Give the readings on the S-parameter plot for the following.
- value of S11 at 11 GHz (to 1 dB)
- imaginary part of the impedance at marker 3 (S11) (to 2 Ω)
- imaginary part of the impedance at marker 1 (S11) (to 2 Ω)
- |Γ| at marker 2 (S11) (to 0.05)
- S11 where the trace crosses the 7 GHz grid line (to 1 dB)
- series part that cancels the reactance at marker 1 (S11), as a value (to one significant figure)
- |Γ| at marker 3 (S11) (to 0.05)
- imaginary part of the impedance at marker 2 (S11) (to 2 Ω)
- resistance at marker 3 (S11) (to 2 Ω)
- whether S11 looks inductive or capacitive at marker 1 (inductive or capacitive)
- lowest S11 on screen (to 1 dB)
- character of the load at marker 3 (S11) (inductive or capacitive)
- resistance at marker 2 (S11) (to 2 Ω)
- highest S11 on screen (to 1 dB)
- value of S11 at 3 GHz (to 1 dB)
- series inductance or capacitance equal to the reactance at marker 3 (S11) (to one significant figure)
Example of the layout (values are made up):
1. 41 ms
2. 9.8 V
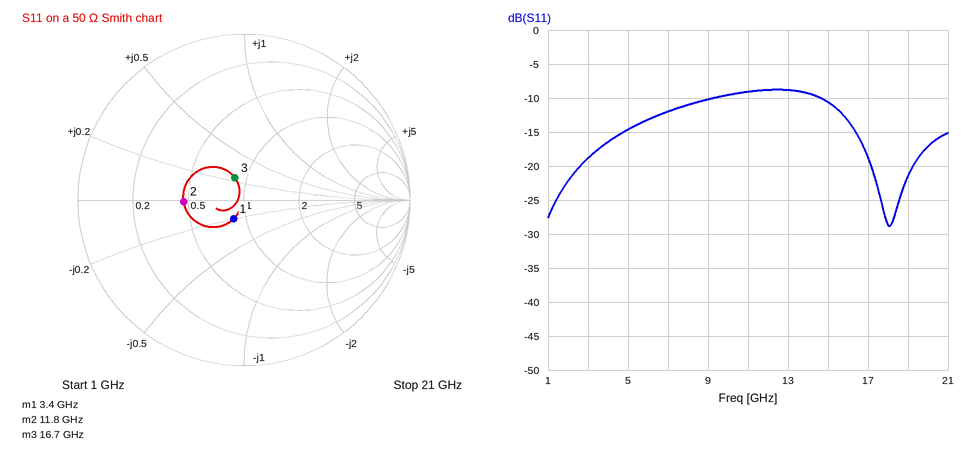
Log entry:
1. -9 dB
2. +12 Ω
3. -10 Ω
4. 0.35
5. -12 dB
6. 500 pH
7. 0.15
8. 0 Ω
9. 44 Ω
10. capacitive
11. -29 dB
12. inductive
13. 24 Ω
14. -9 dB
15. -19 dB
16. 100 pH
